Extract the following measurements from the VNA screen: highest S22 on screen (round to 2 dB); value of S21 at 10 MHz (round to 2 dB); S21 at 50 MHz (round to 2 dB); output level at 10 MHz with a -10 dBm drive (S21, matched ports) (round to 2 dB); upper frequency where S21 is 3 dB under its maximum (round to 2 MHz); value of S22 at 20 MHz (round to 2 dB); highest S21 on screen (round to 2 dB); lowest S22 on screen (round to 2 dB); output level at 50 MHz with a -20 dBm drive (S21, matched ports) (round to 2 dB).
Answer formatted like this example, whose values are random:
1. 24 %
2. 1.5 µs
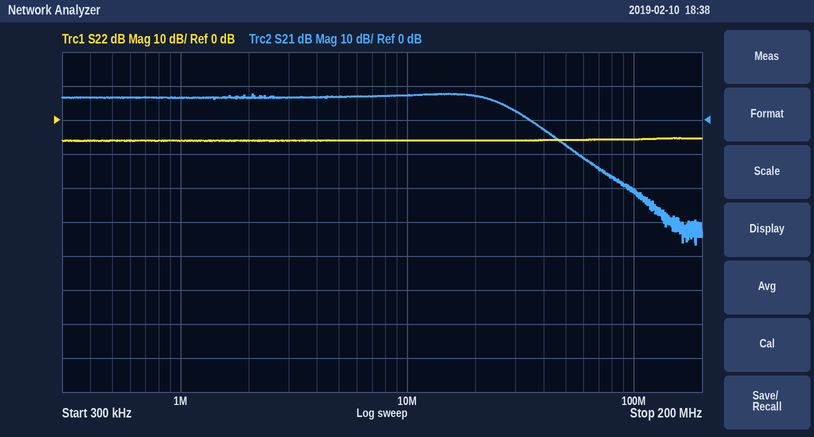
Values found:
1. -6 dB
2. 8 dB
3. -8 dB
4. -2 dBm
5. 26 MHz
6. -6 dB
7. 8 dB
8. -6 dB
9. -28 dBm
